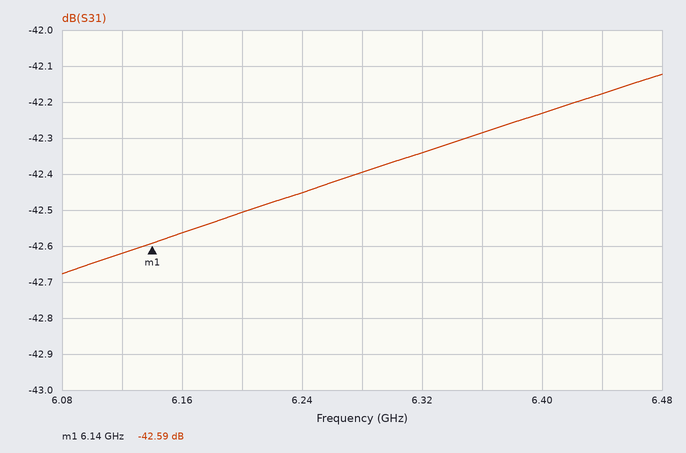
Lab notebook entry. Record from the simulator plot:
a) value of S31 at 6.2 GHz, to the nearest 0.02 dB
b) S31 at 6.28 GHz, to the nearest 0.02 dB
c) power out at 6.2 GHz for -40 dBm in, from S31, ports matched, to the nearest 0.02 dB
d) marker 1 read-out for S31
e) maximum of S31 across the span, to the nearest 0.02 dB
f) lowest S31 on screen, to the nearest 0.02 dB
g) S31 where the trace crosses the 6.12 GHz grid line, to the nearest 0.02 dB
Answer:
-42.50 dB
-42.40 dB
-82.50 dBm
-42.59 dB
-42.12 dB
-42.68 dB
-42.62 dB
